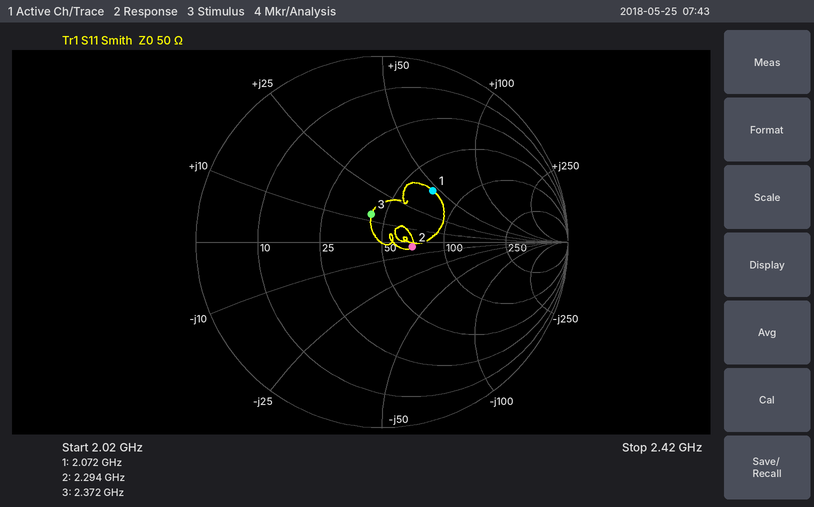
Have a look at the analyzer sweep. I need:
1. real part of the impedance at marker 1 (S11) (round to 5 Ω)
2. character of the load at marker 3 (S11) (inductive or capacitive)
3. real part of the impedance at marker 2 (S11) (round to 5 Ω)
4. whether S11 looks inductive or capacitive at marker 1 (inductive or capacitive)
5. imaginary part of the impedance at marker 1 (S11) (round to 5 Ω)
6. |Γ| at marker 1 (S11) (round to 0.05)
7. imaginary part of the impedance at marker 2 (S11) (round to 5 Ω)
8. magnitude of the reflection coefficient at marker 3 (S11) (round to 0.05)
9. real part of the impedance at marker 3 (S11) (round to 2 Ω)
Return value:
70 Ω
inductive
70 Ω
inductive
+45 Ω
0.40
-5 Ω
0.15
42 Ω
